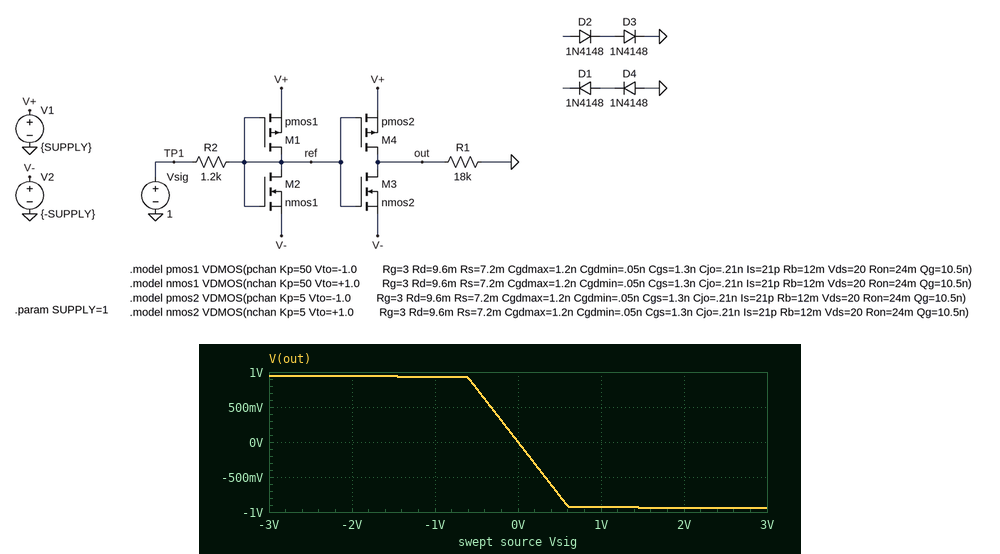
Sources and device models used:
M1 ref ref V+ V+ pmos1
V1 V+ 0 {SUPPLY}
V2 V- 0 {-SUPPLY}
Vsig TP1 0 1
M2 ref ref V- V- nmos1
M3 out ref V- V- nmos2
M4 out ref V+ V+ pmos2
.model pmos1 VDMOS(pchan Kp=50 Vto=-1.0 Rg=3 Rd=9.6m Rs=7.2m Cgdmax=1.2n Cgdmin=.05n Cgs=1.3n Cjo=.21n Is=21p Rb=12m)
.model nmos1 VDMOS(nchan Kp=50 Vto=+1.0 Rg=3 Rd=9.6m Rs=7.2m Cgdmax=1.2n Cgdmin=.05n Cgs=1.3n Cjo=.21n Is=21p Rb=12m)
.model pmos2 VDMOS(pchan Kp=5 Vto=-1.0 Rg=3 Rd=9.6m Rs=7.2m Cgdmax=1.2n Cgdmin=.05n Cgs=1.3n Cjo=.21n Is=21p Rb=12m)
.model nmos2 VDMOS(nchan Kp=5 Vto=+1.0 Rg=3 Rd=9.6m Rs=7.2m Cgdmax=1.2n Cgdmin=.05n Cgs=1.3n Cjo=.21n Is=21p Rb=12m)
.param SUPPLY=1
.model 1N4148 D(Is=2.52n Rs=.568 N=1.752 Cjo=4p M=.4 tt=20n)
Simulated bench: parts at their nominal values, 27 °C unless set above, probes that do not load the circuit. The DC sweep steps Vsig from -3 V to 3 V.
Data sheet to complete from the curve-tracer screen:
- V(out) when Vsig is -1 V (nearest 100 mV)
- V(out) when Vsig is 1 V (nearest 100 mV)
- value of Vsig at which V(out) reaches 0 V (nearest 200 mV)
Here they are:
900 mV
-900 mV
0 V
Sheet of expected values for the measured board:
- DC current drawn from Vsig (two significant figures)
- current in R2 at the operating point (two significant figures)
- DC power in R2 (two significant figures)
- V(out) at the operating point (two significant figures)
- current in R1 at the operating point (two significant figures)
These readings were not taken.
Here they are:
830 µA
830 µA
830 µW
-930 mV
52 µA
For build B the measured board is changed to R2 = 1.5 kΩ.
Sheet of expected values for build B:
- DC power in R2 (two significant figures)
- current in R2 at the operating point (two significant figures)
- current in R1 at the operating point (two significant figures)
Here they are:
670 µW
670 µA
52 µA
